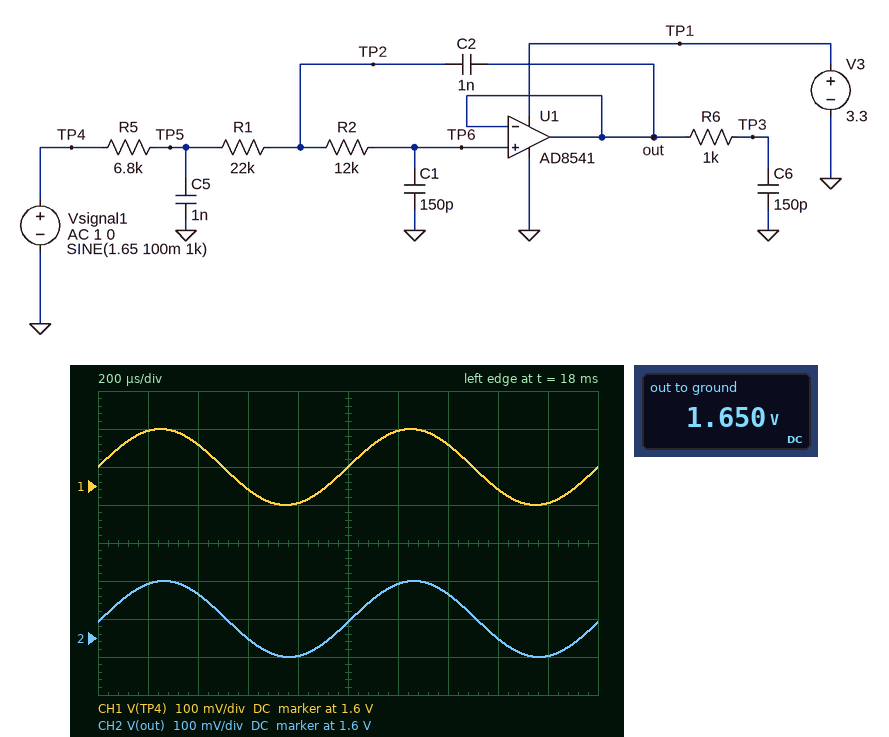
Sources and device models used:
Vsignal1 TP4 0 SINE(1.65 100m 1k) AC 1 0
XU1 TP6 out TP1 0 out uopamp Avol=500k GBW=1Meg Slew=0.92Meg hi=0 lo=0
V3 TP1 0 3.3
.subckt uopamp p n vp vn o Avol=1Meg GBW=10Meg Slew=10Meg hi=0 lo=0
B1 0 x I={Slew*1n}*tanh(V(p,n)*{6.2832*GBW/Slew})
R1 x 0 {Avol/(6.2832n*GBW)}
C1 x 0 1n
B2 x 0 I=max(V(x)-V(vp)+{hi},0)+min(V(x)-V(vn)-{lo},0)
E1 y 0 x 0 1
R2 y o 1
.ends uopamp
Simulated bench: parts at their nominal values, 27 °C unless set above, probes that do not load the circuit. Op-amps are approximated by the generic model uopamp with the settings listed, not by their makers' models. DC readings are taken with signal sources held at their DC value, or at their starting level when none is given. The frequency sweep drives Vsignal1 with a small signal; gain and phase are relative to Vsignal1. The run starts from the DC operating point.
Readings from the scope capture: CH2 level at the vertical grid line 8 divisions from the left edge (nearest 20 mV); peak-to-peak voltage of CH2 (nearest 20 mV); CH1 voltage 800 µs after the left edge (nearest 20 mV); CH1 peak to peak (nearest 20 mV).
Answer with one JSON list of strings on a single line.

["1.60 V", "200 mV", "1.56 V", "200 mV"]
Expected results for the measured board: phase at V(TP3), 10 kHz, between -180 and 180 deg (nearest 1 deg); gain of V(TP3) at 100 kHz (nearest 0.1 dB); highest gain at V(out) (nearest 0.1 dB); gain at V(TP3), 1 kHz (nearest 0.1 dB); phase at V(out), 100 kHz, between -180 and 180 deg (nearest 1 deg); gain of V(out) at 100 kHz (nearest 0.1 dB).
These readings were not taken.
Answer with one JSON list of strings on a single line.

["-50 deg", "-37.4 dB", "0.2 dB", "0 dB", "113 deg", "-37.4 dB"]
